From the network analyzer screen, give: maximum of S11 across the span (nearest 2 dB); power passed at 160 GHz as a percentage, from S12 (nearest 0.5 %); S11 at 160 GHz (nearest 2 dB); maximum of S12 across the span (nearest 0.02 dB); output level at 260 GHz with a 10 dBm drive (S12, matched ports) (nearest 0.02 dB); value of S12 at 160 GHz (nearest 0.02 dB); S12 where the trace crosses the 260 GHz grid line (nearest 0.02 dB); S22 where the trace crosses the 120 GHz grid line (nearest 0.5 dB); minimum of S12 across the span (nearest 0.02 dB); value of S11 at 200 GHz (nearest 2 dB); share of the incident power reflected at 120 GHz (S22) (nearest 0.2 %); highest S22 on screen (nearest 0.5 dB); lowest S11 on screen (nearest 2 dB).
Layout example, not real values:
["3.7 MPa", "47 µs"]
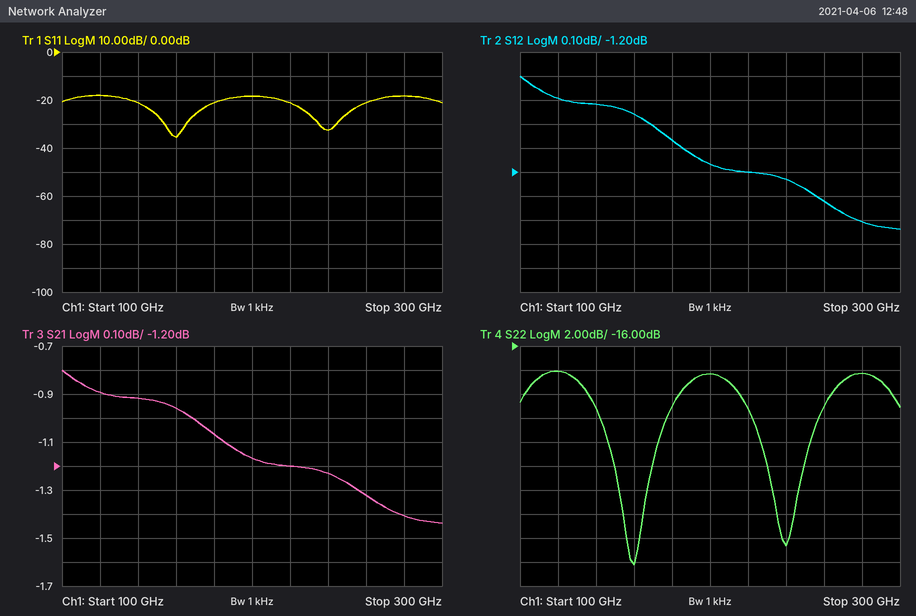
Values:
["-18 dB", "80.0 %", "-36 dB", "-0.80 dB", "8.68 dBm", "-0.96 dB", "-1.32 dB", "-18.0 dB", "-1.44 dB", "-18 dB", "1.6 %", "-18.0 dB", "-36 dB"]
